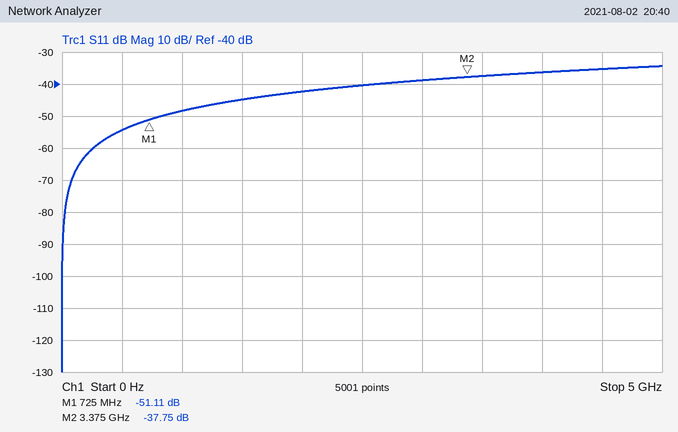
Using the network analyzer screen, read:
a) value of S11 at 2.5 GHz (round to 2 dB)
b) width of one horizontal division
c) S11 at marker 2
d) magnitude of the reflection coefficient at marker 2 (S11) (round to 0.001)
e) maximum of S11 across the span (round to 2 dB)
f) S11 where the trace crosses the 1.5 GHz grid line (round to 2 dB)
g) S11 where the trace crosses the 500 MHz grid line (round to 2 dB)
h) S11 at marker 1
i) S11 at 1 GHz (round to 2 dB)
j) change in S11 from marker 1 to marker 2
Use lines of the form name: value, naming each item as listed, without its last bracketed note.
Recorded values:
value of S11 at 2.5 GHz: -40 dB
width of one horizontal division: 500 MHz
S11 at marker 2: -37.75 dB
magnitude of the reflection coefficient at marker 2 (S11): 0.013
maximum of S11 across the span: -34 dB
S11 where the trace crosses the 1.5 GHz grid line: -44 dB
S11 where the trace crosses the 500 MHz grid line: -54 dB
S11 at marker 1: -51.11 dB
S11 at 1 GHz: -48 dB
change in S11 from marker 1 to marker 2: 13.36 dB
